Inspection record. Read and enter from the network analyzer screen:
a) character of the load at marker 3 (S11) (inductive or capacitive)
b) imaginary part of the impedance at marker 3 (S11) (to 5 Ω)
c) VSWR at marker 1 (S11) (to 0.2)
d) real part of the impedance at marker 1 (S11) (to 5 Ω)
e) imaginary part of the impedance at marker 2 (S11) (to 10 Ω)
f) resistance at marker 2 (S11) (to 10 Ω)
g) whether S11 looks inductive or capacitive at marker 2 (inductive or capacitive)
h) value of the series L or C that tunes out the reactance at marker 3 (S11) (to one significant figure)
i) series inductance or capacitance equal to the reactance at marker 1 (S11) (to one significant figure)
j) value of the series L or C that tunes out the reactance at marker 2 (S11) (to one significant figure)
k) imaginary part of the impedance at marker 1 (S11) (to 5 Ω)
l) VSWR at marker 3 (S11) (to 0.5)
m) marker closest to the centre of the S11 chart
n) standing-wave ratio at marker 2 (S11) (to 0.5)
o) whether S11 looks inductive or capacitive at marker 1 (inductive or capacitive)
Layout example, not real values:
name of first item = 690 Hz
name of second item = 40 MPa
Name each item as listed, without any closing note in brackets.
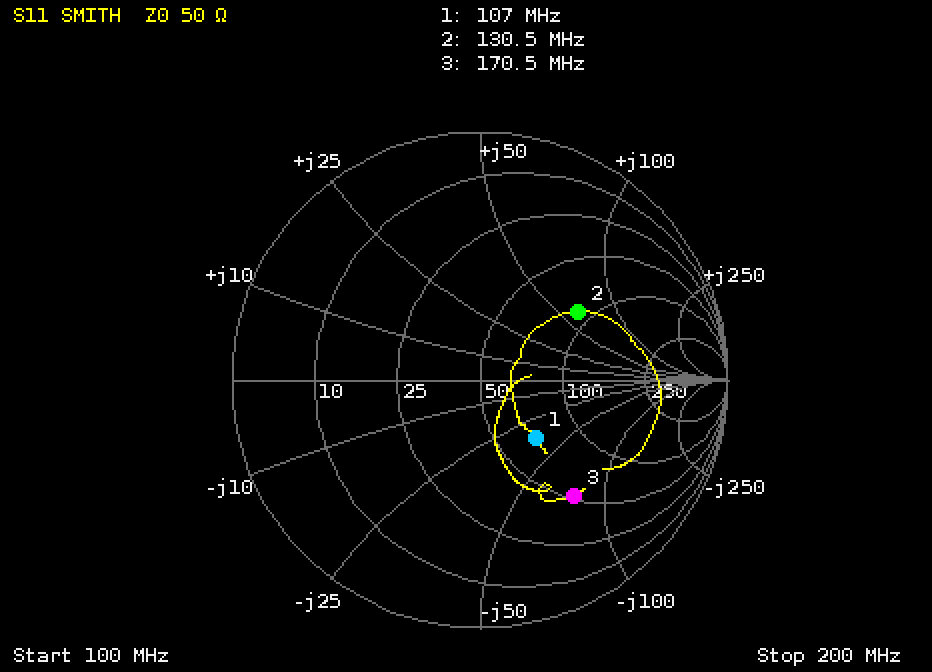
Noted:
character of the load at marker 3 (S11) = capacitive
imaginary part of the impedance at marker 3 (S11) = -75 Ω
VSWR at marker 1 (S11) = 2.0
real part of the impedance at marker 1 (S11) = 70 Ω
imaginary part of the impedance at marker 2 (S11) = +60 Ω
resistance at marker 2 (S11) = 90 Ω
whether S11 looks inductive or capacitive at marker 2 = inductive
value of the series L or C that tunes out the reactance at marker 3 (S11) = 70 nH
series inductance or capacitance equal to the reactance at marker 1 (S11) = 40 pF
value of the series L or C that tunes out the reactance at marker 2 (S11) = 20 pF
imaginary part of the impedance at marker 1 (S11) = -35 Ω
VSWR at marker 3 (S11) = 4.0
marker closest to the centre of the S11 chart = marker 1
standing-wave ratio at marker 2 (S11) = 3.0
whether S11 looks inductive or capacitive at marker 1 = capacitive
